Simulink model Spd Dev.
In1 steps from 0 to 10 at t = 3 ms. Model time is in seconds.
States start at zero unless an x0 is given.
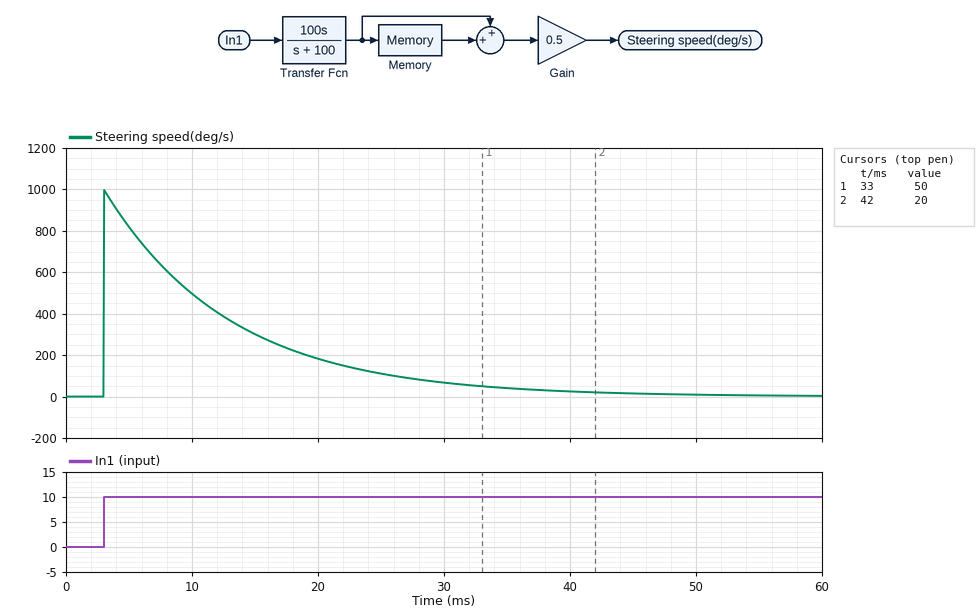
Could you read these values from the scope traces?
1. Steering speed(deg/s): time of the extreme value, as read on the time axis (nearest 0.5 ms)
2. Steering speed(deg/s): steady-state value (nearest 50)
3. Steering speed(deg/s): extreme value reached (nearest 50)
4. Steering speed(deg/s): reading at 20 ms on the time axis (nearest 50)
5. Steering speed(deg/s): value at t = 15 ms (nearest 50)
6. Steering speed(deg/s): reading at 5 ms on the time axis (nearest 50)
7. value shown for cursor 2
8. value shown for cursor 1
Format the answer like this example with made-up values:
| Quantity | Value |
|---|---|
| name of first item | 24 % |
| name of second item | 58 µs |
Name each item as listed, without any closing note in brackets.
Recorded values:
| Quantity | Value |
|---|---|
| Steering speed(deg/s): time of the extreme value, as read on the time axis | 3.0 ms |
| Steering speed(deg/s): steady-state value | 0 |
| Steering speed(deg/s): extreme value reached | 1000 |
| Steering speed(deg/s): reading at 20 ms on the time axis | 200 |
| Steering speed(deg/s): value at t = 15 ms | 300 |
| Steering speed(deg/s): reading at 5 ms on the time axis | 800 |
| value shown for cursor 2 | 20 |
| value shown for cursor 1 | 50 |
